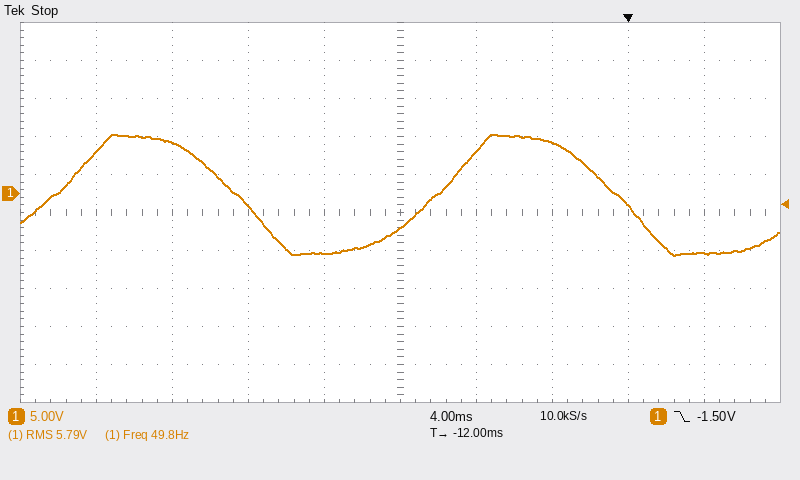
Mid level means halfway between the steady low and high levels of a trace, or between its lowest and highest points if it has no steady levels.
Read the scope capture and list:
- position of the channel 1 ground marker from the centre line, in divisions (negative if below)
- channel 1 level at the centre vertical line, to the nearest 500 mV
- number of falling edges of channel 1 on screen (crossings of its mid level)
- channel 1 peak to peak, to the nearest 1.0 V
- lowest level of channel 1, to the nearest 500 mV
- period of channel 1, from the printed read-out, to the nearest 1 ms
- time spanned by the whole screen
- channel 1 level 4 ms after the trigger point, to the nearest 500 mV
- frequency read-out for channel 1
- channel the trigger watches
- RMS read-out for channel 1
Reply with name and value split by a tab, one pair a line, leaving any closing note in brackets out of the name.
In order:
position of the channel 1 ground marker from the centre line, in divisions	+0.5 div
channel 1 level at the centre vertical line, to the nearest 500 mV	-4.5 V
number of falling edges of channel 1 on screen	2
channel 1 peak to peak, to the nearest 1.0 V	16.0 V
lowest level of channel 1, to the nearest 500 mV	-8.0 V
period of channel 1, from the printed read-out, to the nearest 1 ms	20 ms
time spanned by the whole screen	40 ms
channel 1 level 4 ms after the trigger point, to the nearest 500 mV	-8.0 V
frequency read-out for channel 1	49.8 Hz
channel the trigger watches	channel 1
RMS read-out for channel 1	5.79 V
